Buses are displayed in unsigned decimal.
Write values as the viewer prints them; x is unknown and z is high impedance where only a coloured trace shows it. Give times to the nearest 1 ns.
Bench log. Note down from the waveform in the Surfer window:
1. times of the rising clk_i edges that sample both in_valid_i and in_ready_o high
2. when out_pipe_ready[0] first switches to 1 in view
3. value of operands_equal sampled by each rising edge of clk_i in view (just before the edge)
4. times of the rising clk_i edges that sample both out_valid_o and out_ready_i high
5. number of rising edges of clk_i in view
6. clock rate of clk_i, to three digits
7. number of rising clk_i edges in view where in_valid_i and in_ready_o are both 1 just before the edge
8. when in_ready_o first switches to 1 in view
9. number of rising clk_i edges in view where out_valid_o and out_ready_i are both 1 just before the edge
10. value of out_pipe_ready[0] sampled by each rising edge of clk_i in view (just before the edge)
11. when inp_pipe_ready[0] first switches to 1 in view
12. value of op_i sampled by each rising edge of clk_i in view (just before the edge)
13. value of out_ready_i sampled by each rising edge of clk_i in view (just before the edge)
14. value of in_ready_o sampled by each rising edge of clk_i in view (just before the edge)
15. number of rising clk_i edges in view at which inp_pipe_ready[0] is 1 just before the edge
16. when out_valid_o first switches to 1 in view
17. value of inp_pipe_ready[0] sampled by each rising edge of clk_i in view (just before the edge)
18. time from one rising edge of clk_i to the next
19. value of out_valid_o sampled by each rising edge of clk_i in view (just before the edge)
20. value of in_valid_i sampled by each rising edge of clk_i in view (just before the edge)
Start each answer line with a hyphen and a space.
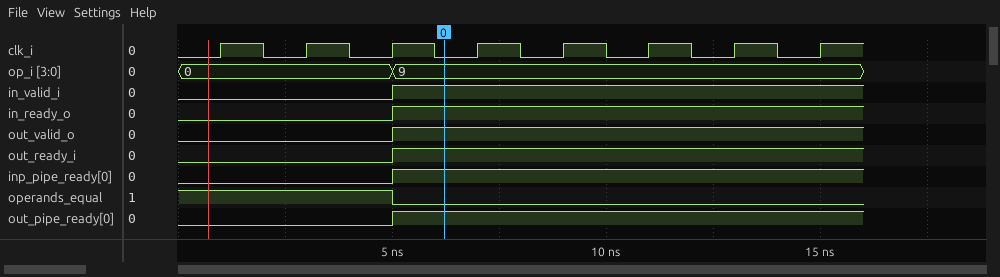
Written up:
- 7 ns, 9 ns, 11 ns, 13 ns, 15 ns
- 5 ns
- 1 1 1 0 0 0 0 0
- 7 ns, 9 ns, 11 ns, 13 ns, 15 ns
- 8
- 500 MHz
- 5
- 5 ns
- 5
- 0 0 0 1 1 1 1 1
- 5 ns
- 0, 0, 0, 9, 9, 9, 9, 9
- 0 0 0 1 1 1 1 1
- 0 0 0 1 1 1 1 1
- 5
- 5 ns
- 0 0 0 1 1 1 1 1
- 2 ns
- 0 0 0 1 1 1 1 1
- 0 0 0 1 1 1 1 1
